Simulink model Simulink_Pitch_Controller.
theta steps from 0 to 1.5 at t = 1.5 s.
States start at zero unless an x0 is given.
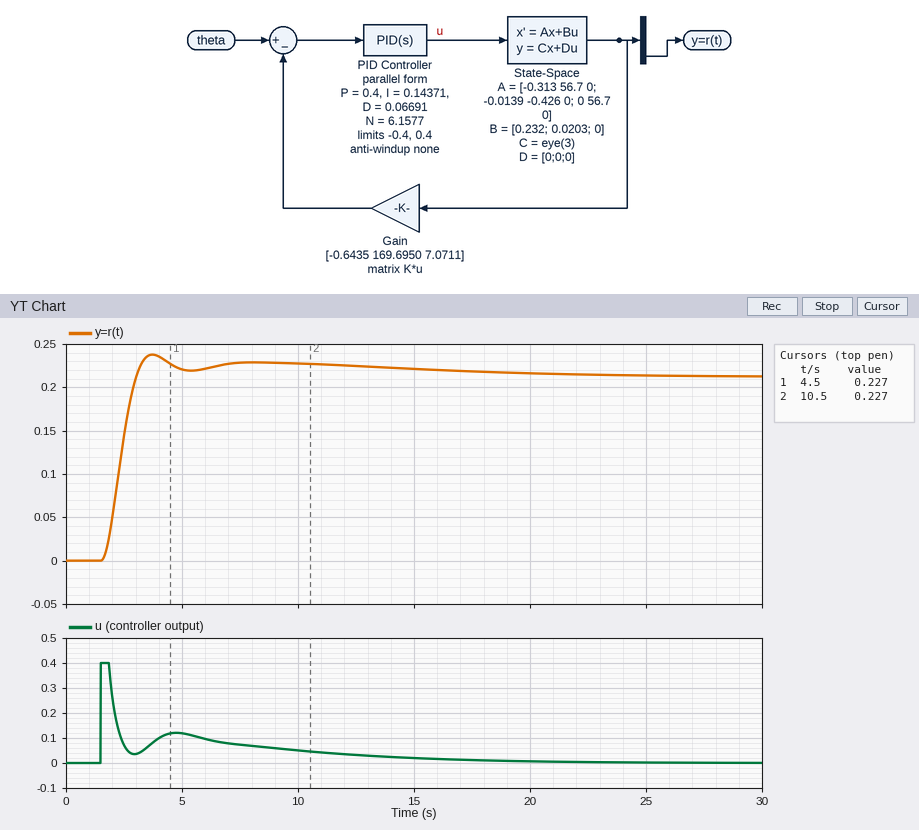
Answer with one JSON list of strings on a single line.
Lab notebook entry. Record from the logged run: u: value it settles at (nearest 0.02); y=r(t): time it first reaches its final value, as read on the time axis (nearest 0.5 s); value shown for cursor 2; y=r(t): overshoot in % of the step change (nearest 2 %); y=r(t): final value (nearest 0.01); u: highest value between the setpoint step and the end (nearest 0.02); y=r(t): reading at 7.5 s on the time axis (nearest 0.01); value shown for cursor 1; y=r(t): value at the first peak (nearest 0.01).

["0.00", "3.0 s", "0.227", "12 %", "0.21", "0.40", "0.23", "0.227", "0.24"]
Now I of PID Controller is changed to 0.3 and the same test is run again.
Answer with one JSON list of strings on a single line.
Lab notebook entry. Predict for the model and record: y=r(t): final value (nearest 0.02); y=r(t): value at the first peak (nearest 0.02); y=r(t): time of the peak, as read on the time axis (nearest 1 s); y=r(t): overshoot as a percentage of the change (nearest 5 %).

["0.22", "0.26", "4 s", "25 %"]
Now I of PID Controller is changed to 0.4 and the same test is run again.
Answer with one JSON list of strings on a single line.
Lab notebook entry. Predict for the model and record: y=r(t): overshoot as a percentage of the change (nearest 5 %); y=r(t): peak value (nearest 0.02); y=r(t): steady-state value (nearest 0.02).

["30 %", "0.28", "0.22"]
